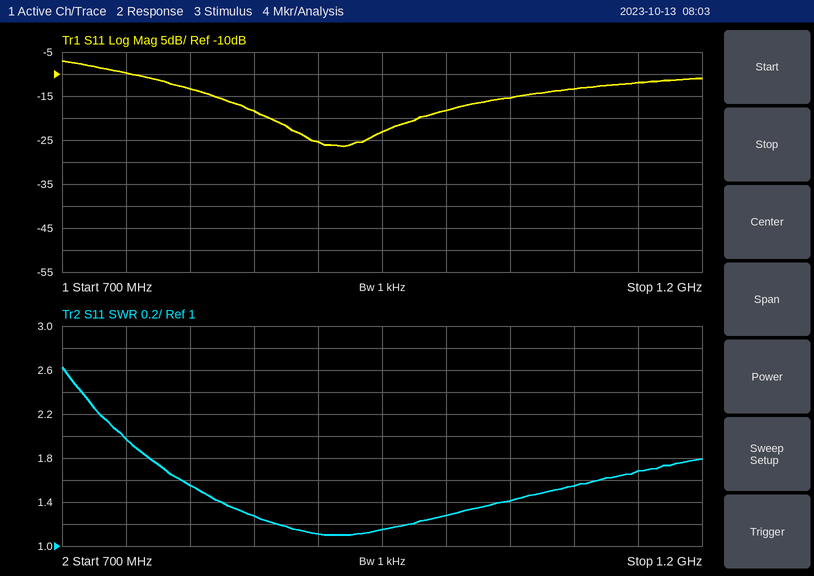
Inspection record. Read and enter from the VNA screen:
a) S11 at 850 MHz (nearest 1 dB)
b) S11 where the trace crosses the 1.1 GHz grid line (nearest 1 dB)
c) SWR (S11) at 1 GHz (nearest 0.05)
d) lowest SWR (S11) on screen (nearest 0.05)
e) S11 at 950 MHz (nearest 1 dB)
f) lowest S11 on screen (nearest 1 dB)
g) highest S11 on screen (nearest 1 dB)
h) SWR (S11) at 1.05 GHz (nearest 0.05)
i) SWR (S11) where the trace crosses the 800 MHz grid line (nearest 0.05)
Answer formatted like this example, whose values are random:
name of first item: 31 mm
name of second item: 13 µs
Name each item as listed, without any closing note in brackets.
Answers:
S11 at 850 MHz: -18 dB
S11 where the trace crosses the 1.1 GHz grid line: -13 dB
SWR (S11) at 1 GHz: 1.30
lowest SWR (S11) on screen: 1.10
S11 at 950 MHz: -23 dB
lowest S11 on screen: -26 dB
highest S11 on screen: -7 dB
SWR (S11) at 1.05 GHz: 1.40
SWR (S11) where the trace crosses the 800 MHz grid line: 1.55
